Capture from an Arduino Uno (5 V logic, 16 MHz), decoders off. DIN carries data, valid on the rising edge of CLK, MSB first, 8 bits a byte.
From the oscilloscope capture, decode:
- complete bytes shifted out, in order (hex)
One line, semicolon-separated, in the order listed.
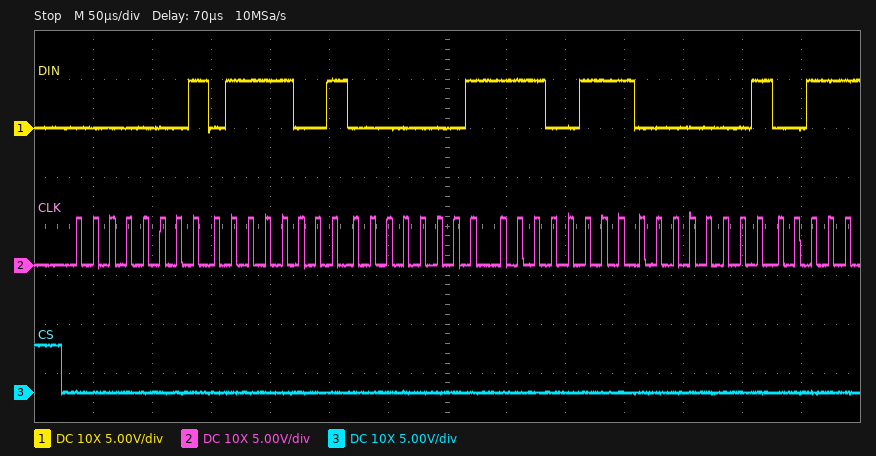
01 79 01 E7 01
